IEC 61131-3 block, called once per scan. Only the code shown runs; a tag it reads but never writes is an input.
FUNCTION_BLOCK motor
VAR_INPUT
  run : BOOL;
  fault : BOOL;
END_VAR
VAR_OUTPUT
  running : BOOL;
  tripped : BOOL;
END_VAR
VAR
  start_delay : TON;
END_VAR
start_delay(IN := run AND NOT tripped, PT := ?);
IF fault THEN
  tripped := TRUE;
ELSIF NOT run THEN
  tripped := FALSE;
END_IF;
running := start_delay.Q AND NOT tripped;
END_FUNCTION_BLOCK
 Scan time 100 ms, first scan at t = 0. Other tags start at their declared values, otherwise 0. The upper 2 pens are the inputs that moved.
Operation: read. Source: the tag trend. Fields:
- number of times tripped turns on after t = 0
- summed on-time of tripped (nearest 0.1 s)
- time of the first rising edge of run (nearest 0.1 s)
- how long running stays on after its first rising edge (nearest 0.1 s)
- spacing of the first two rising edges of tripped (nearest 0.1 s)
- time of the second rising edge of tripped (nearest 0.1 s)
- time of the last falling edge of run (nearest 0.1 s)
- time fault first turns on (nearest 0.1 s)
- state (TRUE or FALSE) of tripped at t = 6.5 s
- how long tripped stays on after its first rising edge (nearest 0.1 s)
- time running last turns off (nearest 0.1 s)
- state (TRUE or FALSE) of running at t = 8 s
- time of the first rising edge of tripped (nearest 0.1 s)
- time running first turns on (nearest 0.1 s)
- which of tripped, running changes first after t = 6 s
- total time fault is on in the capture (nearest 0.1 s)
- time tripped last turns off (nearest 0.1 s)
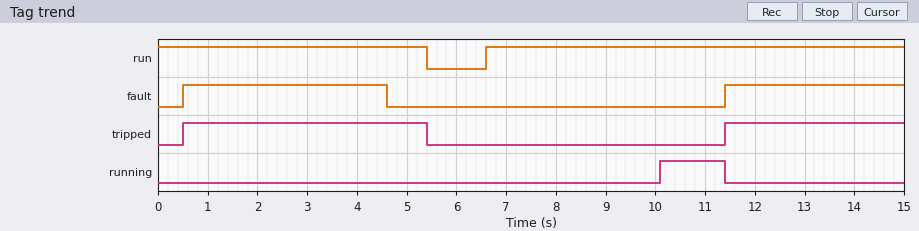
2
8.5 s
6.6 s
1.3 s
10.9 s
11.4 s
5.4 s
0.5 s
FALSE
4.9 s
11.4 s
FALSE
0.5 s
10.1 s
running
7.7 s
5.4 s
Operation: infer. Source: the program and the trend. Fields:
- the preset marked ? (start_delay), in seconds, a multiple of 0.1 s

3.5 s
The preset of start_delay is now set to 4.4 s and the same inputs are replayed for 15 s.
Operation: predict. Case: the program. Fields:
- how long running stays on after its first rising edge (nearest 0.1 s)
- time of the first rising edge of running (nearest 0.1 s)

0.4 s
11.0 s
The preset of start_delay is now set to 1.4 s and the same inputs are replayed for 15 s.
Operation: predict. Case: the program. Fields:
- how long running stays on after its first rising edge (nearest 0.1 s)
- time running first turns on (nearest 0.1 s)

3.4 s
8.0 s
